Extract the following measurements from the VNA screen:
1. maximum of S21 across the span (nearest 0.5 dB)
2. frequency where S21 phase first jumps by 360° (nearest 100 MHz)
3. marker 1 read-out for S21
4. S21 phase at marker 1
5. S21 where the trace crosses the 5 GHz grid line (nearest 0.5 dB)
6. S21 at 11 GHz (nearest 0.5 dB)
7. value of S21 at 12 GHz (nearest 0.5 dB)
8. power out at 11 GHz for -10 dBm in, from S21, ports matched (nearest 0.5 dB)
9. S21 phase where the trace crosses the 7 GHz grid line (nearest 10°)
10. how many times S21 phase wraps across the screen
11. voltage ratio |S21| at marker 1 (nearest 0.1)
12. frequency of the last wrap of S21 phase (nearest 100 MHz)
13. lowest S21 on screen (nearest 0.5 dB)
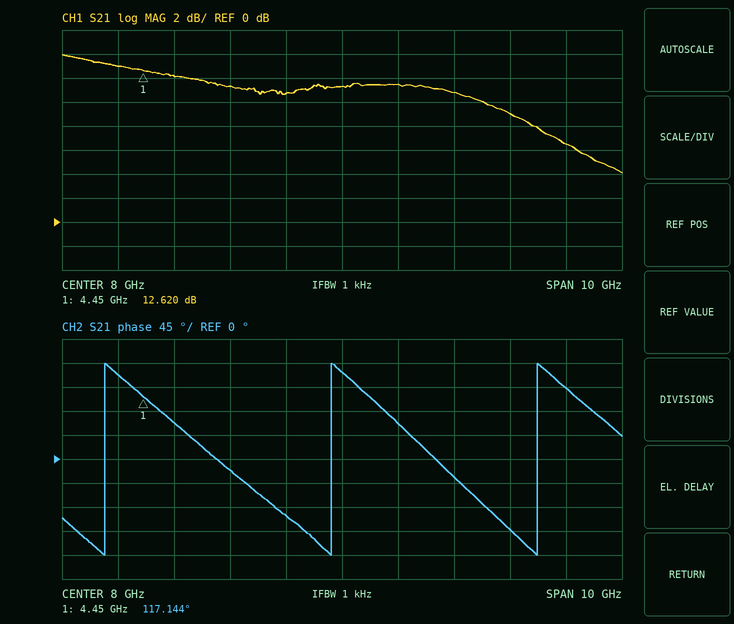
14.0 dB
3.8 GHz
12.620 dB
117.144°
12.0 dB
9.0 dB
6.5 dB
-1.0 dBm
-110°
3
4.3
11.5 GHz
4.0 dB
